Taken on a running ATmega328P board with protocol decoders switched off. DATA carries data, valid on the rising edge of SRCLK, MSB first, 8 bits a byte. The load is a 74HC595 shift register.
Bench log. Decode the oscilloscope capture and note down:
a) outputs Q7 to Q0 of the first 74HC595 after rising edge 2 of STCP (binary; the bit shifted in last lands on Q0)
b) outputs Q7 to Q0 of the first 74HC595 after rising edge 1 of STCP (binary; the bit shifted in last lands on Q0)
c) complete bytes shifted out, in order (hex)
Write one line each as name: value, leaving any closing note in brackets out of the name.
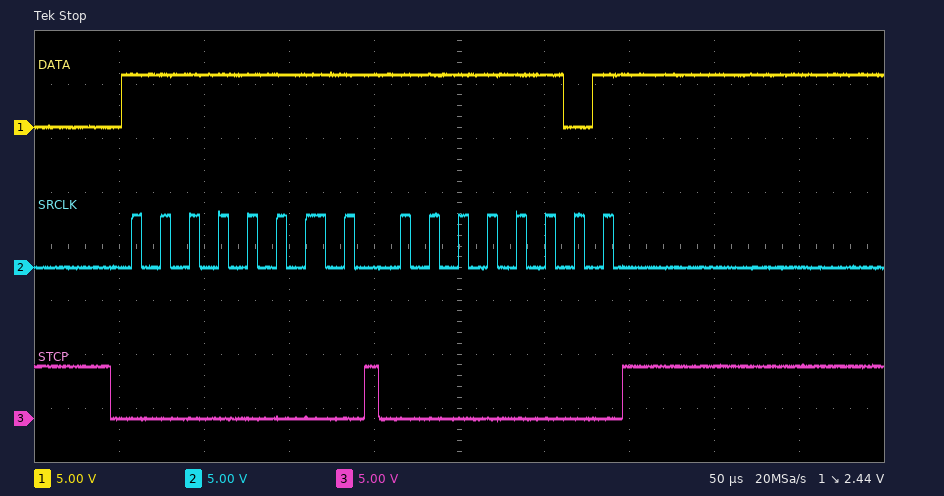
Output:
outputs Q7 to Q0 of the first 74HC595 after rising edge 2 of STCP: 11111101
outputs Q7 to Q0 of the first 74HC595 after rising edge 1 of STCP: 11111111
complete bytes shifted out, in order: FF FD
